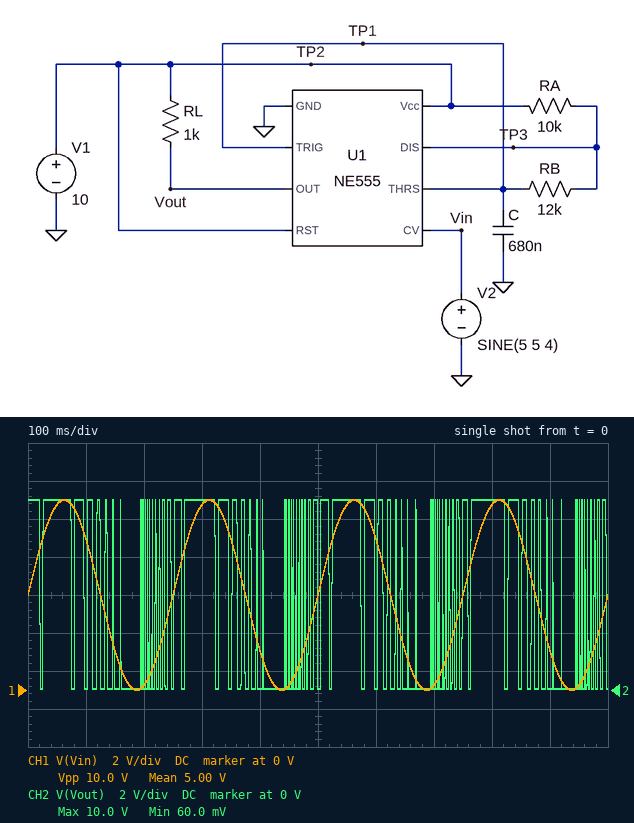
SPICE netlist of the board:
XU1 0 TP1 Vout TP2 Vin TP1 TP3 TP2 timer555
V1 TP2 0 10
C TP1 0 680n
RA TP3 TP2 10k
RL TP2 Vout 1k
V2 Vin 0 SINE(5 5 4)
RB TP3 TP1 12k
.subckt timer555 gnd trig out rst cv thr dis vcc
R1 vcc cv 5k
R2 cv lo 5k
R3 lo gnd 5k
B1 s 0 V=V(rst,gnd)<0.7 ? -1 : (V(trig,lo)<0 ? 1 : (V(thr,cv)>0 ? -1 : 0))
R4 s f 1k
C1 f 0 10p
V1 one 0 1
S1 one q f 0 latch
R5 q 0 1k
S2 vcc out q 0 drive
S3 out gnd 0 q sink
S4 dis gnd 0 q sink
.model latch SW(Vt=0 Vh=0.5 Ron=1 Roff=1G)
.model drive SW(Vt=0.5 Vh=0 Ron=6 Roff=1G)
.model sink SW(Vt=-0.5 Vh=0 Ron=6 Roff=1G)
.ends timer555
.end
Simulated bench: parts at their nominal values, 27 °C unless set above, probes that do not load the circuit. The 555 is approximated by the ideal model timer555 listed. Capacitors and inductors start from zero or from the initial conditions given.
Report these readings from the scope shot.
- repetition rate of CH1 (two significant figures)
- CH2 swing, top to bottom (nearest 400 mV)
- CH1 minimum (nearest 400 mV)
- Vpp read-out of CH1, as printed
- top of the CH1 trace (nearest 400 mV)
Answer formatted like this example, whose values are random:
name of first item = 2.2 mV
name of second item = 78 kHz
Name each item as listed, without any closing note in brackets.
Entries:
repetition rate of CH1 = 4.0 Hz
CH2 swing, top to bottom = 10.0 V
CH1 minimum = 0 V
Vpp read-out of CH1, as printed = 10.0 V
top of the CH1 trace = 10.0 V
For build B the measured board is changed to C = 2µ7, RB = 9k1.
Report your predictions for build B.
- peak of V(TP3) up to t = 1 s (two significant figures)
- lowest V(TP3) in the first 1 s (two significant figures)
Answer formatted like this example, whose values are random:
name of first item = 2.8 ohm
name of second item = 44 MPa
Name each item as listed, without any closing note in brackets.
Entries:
peak of V(TP3) up to t = 1 s = 9.5 V
lowest V(TP3) in the first 1 s = 6.1 mV
